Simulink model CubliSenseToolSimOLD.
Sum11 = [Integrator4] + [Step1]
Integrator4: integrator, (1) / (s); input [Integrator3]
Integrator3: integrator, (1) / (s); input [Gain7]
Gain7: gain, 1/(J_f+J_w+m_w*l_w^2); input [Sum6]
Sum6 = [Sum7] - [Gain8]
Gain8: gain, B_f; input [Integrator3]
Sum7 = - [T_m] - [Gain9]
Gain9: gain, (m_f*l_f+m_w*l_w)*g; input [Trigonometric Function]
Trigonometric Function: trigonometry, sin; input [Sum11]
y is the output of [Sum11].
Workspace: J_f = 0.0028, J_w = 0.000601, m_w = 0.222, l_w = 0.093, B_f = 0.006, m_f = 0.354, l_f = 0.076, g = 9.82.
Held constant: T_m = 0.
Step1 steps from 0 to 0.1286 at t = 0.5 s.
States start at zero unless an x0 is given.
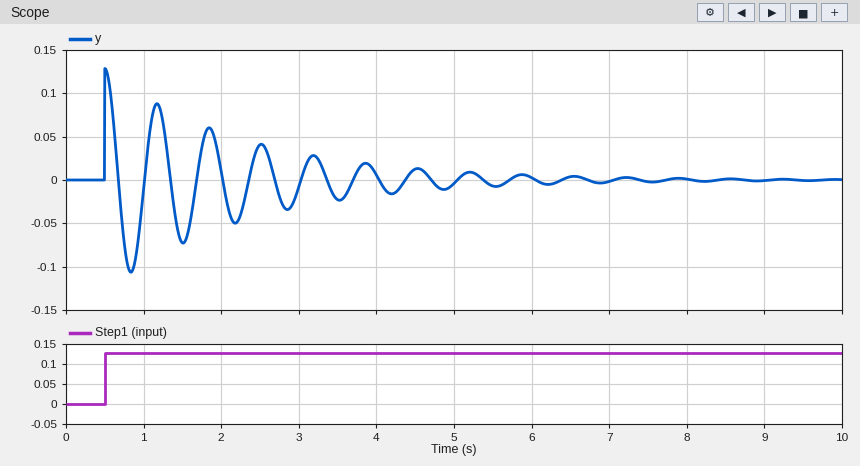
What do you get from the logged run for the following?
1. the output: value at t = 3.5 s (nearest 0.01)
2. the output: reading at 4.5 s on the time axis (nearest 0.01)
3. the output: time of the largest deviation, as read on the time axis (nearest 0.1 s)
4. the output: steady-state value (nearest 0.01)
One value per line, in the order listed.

-0.02
0.01
0.5 s
0.00
